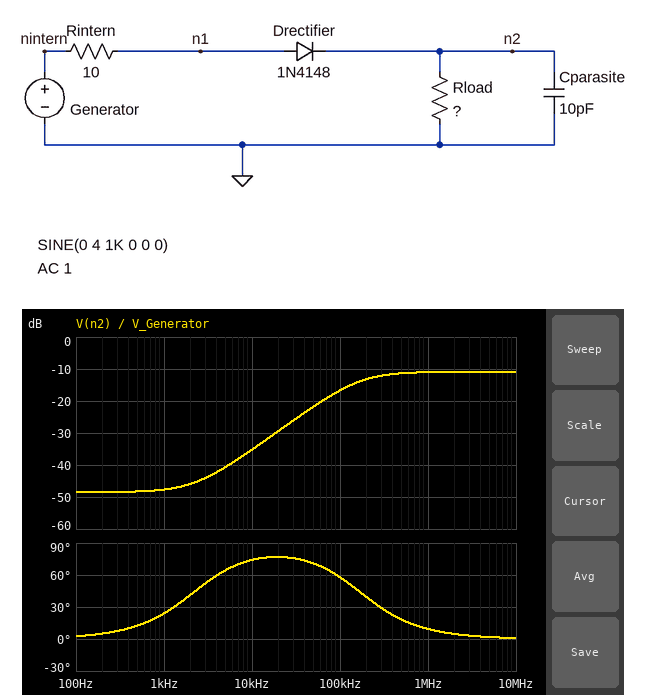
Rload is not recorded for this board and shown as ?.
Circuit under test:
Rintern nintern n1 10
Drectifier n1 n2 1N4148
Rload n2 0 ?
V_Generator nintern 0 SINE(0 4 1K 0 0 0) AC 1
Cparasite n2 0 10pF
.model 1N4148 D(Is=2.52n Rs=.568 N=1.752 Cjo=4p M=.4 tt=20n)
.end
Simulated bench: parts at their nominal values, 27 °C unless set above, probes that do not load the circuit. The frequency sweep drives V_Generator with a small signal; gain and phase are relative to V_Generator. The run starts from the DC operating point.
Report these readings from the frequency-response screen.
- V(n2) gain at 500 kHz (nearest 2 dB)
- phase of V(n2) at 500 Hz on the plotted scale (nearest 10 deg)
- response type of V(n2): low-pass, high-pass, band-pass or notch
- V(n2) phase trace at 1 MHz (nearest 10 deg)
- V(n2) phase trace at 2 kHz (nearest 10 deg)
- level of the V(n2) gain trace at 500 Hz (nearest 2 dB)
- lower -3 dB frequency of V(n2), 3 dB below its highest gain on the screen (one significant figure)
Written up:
-12 dB
10 deg
high-pass
10 deg
40 deg
-48 dB
200 kHz
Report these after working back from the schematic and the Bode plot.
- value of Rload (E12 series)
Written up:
68 kΩ
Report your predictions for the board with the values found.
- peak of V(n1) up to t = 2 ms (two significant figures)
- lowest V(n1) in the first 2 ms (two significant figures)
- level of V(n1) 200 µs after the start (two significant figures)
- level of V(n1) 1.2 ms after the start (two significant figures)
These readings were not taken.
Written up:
4.0 V
-4.0 V
3.8 V
3.8 V
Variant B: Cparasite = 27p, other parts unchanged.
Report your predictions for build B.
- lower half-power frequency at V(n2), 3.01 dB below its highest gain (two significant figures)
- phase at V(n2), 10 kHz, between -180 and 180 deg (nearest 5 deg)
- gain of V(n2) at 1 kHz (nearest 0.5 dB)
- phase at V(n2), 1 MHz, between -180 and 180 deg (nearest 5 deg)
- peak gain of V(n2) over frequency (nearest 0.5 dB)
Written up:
76 kHz
70 deg
-47.5 dB
5 deg
-18.0 dB
